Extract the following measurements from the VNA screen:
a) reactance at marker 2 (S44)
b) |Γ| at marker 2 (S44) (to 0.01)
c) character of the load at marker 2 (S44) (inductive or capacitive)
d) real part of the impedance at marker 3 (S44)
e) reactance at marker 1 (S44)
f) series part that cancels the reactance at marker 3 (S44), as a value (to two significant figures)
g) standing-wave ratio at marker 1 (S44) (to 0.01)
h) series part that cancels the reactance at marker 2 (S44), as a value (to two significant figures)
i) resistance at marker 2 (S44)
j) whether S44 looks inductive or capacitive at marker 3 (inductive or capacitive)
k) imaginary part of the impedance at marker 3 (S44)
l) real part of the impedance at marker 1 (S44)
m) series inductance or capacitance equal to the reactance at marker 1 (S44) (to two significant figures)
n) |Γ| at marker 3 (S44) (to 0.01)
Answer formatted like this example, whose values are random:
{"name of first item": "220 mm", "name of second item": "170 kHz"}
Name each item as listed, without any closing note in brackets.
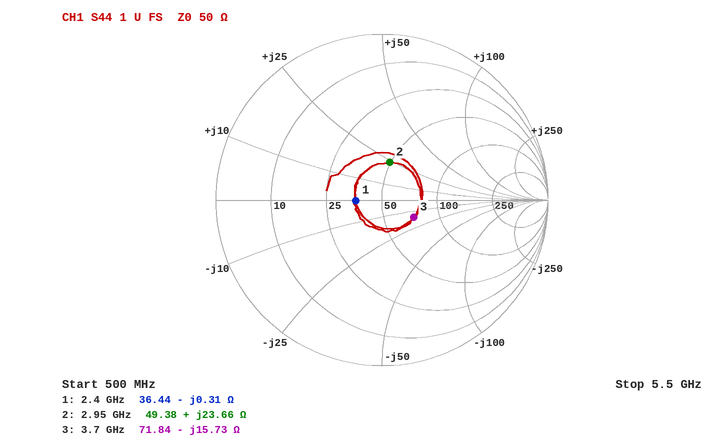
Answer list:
{"reactance at marker 2": "+23.66 Ω", "|Γ| at marker 2 (S44)": "0.23", "character of the load at marker 2 (S44)": "inductive", "real part of the impedance at marker 3": "71.84 Ω", "reactance at marker 1": "-0.31 Ω", "series part that cancels the reactance at marker 3 (S44), as a value": "680 pH", "standing-wave ratio at marker 1 (S44)": "1.37", "series part that cancels the reactance at marker 2 (S44), as a value": "2.3 pF", "resistance at marker 2": "49.38 Ω", "whether S44 looks inductive or capacitive at marker 3": "capacitive", "imaginary part of the impedance at marker 3": "-15.73 Ω", "real part of the impedance at marker 1": "36.44 Ω", "series inductance or capacitance equal to the reactance at marker 1 (S44)": "210 pF", "|Γ| at marker 3 (S44)": "0.22"}
